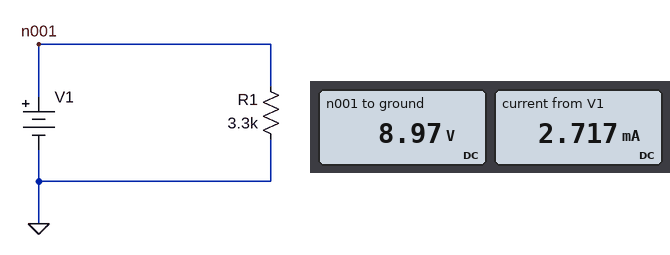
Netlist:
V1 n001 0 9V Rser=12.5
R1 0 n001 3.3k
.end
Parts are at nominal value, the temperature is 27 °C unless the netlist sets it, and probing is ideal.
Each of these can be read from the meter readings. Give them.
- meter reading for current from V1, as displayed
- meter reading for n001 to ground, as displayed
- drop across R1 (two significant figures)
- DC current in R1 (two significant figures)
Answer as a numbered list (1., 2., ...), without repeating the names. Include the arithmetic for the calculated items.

1. 2.717 mA
2. 8.97 V
3. 8.97 V = 9.0 V
4. (8.97 V) / 3.3 kΩ = 2.7 mA
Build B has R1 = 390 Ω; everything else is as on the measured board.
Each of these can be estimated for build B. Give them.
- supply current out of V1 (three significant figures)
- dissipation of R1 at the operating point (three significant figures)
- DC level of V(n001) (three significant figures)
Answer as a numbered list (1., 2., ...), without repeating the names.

1. 22.4 mA
2. 195 mW
3. 8.72 V
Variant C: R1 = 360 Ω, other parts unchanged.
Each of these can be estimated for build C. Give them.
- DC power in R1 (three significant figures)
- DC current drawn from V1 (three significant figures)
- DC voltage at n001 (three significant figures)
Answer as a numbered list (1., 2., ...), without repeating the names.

1. 210 mW
2. 24.2 mA
3. 8.70 V
